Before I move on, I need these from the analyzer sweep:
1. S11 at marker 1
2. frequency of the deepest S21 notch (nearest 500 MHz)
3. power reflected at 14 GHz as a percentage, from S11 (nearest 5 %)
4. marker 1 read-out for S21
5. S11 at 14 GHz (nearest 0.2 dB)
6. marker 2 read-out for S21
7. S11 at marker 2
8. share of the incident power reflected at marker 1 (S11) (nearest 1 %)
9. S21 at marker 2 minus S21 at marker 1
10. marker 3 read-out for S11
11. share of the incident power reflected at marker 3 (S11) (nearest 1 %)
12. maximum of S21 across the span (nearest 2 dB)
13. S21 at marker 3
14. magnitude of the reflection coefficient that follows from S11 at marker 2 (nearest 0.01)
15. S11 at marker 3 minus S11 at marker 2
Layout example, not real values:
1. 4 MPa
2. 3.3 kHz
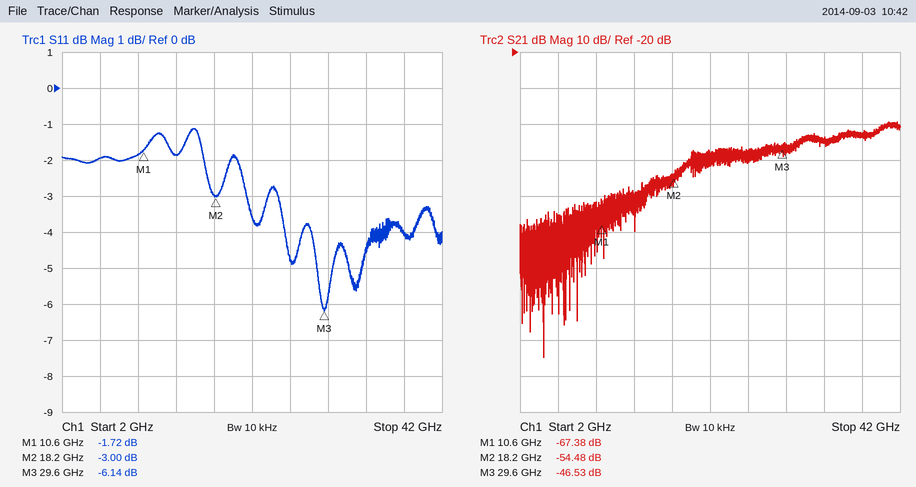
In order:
1. -1.72 dB
2. 4.5 GHz
3. 65 %
4. -67.38 dB
5. -1.8 dB
6. -54.48 dB
7. -3.00 dB
8. 67 %
9. 12.90 dB
10. -6.14 dB
11. 24 %
12. -40 dB
13. -46.53 dB
14. 0.71
15. -3.14 dB
